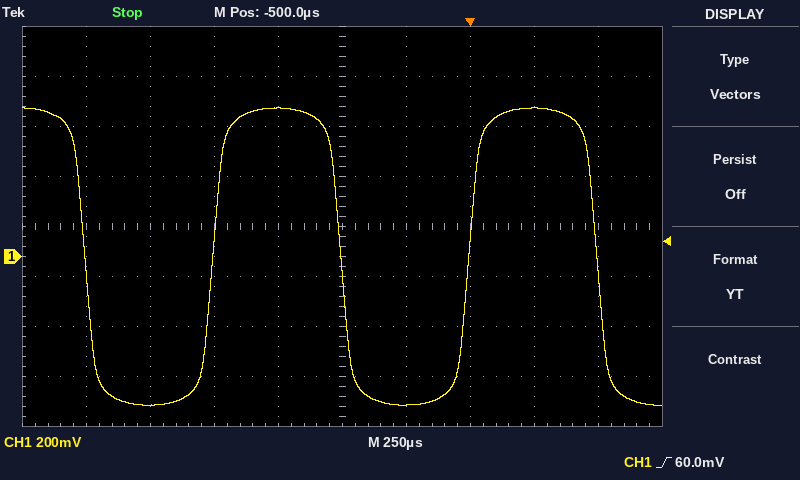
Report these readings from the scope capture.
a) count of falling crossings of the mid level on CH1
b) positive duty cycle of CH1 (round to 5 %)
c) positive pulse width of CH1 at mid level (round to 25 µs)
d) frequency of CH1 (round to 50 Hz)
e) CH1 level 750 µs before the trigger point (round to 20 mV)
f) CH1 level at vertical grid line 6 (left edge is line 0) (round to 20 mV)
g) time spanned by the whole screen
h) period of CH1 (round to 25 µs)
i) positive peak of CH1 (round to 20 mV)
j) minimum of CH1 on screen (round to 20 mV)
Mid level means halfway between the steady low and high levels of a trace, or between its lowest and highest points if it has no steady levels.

3
50 %
500 µs
1.00 kHz
600 mV
-600 mV
2.5 ms
1.000 ms
600 mV
-600 mV
